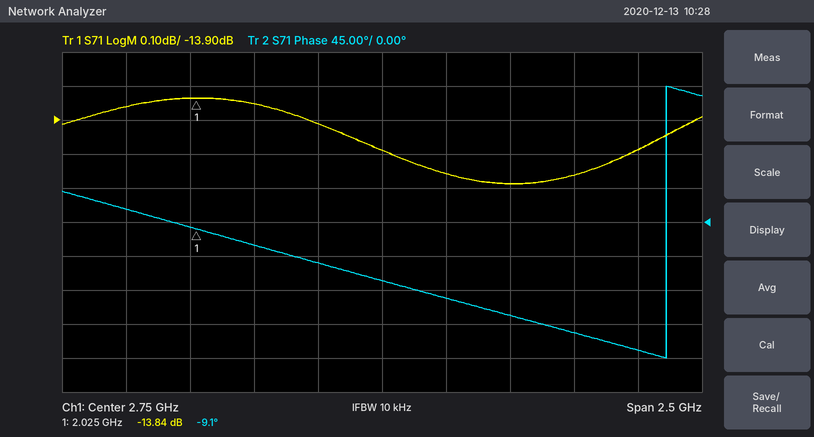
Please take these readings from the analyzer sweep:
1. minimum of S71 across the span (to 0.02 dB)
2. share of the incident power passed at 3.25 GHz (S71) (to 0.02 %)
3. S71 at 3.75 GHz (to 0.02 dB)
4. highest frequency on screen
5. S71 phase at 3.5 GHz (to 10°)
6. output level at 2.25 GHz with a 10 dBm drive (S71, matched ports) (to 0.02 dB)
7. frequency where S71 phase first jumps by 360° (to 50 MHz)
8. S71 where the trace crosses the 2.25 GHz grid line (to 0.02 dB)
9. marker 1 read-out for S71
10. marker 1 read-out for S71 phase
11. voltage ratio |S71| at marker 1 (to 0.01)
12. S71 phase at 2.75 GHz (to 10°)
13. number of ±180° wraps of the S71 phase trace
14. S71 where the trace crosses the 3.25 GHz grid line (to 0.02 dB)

-14.08 dB
3.90 %
-13.98 dB
4 GHz
-150°
-3.86 dBm
3.85 GHz
-13.86 dB
-13.84 dB
-9.1°
0.20
-80°
1
-14.08 dB
